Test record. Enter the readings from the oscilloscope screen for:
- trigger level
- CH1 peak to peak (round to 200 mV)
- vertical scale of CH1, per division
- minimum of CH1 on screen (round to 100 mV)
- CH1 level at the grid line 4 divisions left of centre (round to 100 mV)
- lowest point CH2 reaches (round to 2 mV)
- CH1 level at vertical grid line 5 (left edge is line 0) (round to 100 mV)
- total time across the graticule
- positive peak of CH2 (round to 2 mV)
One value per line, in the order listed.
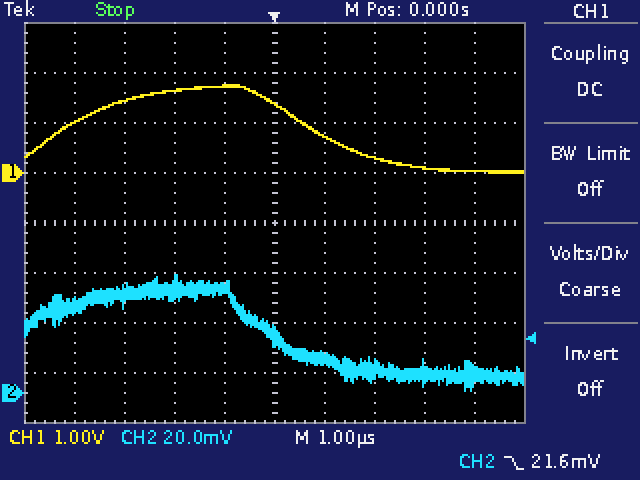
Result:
21.6 mV
1.8 V
1 V
0.0 V
1.0 V
0 mV
1.4 V
10 µs
48 mV
